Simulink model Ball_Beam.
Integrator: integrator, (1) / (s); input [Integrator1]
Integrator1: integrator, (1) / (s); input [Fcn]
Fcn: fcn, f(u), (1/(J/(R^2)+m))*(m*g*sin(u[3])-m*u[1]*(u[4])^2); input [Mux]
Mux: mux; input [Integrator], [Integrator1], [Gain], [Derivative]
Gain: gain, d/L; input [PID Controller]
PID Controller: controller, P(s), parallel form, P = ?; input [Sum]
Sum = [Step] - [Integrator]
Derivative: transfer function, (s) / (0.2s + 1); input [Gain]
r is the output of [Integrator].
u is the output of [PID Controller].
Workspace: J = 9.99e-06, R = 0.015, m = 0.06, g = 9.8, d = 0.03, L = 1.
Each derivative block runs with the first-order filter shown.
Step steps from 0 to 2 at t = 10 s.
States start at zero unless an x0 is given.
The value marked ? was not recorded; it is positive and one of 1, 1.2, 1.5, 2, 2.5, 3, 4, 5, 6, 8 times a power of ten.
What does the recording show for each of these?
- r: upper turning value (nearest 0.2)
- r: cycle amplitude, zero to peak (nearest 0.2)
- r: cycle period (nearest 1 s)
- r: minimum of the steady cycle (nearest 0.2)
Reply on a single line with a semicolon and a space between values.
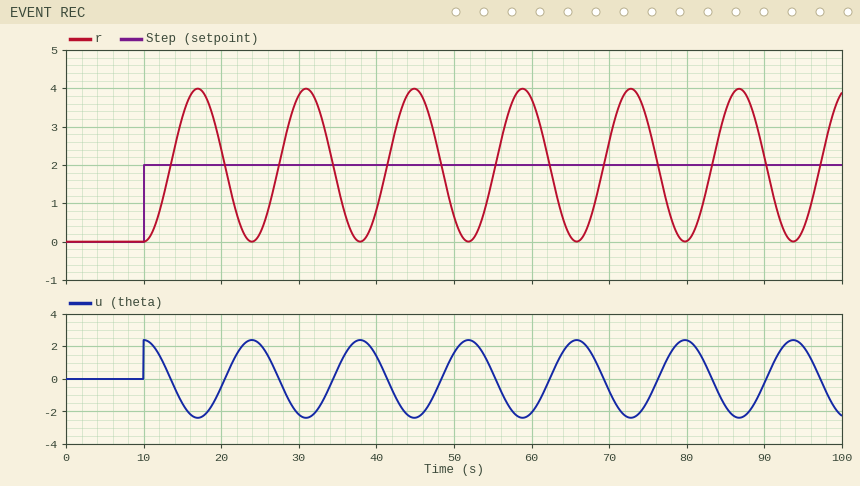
4.0; 2.0; 14 s; 0.0
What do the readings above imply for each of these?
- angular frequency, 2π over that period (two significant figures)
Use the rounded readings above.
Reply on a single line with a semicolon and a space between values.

0.45 rad/s
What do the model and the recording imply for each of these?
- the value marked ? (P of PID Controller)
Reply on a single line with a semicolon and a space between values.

1.2
